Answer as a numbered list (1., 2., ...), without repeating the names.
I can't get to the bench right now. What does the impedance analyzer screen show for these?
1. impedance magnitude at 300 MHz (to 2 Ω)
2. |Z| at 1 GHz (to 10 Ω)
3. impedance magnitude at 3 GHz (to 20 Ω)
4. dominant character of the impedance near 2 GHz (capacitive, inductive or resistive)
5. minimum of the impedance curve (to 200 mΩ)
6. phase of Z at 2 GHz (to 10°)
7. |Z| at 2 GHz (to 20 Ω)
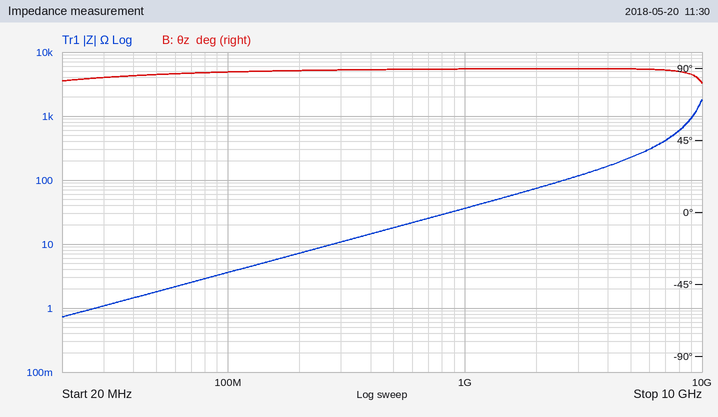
1. 10 Ω
2. 40 Ω
3. 120 Ω
4. inductive
5. 800 mΩ
6. 90°
7. 80 Ω
